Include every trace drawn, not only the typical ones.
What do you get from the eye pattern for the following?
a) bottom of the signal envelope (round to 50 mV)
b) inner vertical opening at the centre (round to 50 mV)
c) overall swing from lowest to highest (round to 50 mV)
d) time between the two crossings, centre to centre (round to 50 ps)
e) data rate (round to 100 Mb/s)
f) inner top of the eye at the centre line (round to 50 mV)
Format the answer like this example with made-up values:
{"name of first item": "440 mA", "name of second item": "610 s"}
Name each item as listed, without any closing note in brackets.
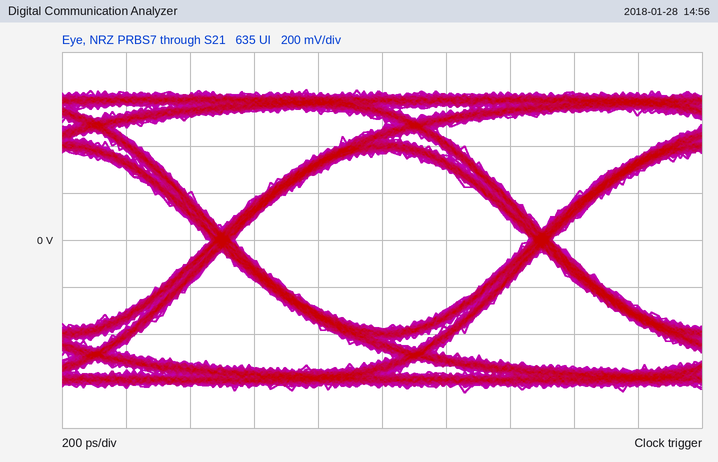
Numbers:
{"bottom of the signal envelope": "-650 mV", "inner vertical opening at the centre": "750 mV", "overall swing from lowest to highest": "1.30 V", "time between the two crossings, centre to centre": "1.00 ns", "data rate": "1.0 Gb/s", "inner top of the eye at the centre line": "350 mV"}
